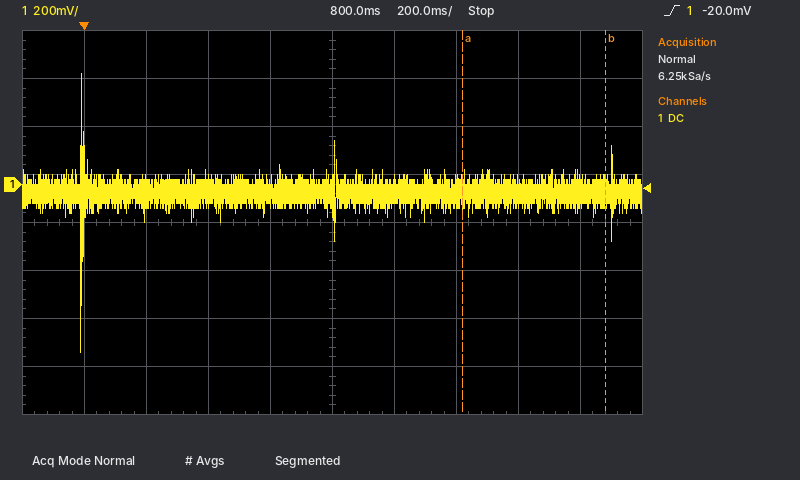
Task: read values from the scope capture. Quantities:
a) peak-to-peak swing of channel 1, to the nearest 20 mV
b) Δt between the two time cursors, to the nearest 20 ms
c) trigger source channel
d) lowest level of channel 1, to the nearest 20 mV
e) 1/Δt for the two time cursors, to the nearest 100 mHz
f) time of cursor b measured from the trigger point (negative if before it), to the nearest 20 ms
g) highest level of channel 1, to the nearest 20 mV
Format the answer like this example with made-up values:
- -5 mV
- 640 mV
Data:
- 1.16 V
- 460 ms
- channel 1
- -700 mV
- 2.2 Hz
- +1.68 s
- 460 mV
